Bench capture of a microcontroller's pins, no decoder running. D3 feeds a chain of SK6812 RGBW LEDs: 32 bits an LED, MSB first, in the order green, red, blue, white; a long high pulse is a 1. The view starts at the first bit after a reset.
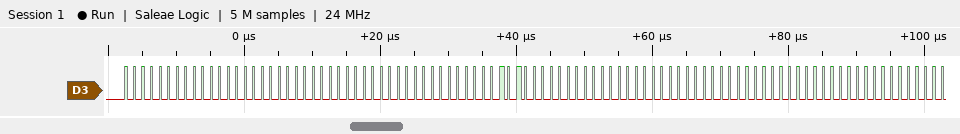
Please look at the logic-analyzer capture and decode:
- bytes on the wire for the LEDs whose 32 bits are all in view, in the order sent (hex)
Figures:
00 00 00 00 00 0A 00 00 00 00 00 00
